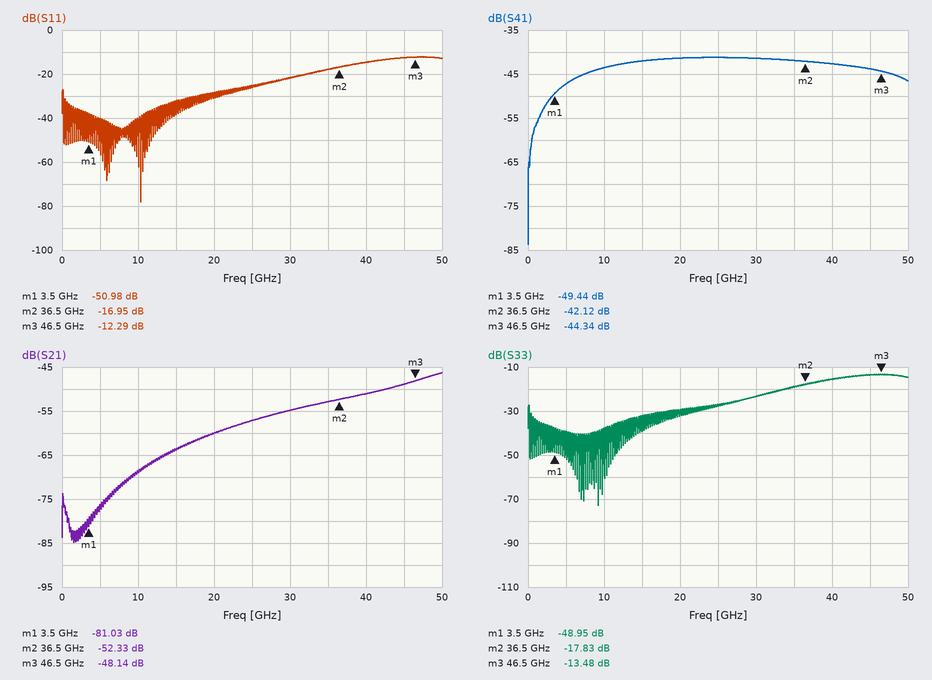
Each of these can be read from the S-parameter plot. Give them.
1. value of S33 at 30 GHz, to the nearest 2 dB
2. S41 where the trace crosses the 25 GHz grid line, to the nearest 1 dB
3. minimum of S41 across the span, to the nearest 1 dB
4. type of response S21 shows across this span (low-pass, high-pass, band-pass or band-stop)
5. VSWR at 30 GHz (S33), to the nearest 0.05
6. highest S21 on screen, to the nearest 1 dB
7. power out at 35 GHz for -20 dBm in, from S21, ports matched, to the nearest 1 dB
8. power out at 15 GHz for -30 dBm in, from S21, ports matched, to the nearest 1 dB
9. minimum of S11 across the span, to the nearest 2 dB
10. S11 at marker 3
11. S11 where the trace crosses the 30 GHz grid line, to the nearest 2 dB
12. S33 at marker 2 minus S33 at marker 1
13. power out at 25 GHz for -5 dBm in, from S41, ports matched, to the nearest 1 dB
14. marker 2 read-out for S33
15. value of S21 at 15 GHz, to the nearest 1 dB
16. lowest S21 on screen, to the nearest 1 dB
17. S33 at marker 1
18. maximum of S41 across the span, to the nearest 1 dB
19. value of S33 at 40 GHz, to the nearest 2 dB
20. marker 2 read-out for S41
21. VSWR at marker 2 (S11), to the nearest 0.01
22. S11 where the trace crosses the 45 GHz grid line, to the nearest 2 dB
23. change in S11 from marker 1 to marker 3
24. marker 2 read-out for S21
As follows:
-24 dB
-41 dB
-84 dB
high-pass
1.15
-46 dB
-73 dBm
-94 dBm
-78 dB
-12.29 dB
-22 dB
31.12 dB
-46 dBm
-17.83 dB
-64 dB
-85 dB
-48.95 dB
-41 dB
-16 dB
-42.12 dB
1.33
-12 dB
38.69 dB
-52.33 dB
